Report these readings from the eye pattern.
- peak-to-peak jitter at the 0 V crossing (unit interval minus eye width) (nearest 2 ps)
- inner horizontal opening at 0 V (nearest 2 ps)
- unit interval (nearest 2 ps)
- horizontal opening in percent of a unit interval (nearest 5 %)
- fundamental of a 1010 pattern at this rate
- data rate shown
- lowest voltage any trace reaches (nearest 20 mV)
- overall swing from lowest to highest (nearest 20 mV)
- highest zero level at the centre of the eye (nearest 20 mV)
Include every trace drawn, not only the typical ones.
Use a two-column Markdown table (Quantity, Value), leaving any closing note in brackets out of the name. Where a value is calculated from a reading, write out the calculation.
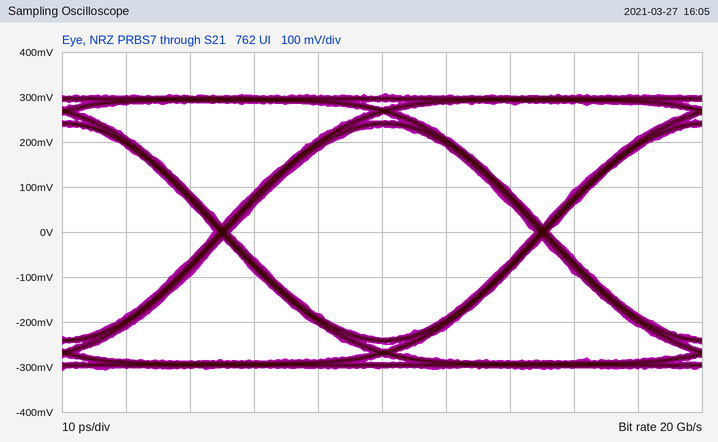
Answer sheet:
| Quantity | Value |
|---|---|
| peak-to-peak jitter at the 0 V crossing (unit interval minus eye width) | 2 ps |
| inner horizontal opening at 0 V | 48 ps |
| unit interval | 50 ps |
| horizontal opening in percent of a unit interval | 48 ps / 50 ps ≈ 96.0 %, so 95 % to the nearest 5 % |
| fundamental of a 1010 pattern at this rate | 10 GHz |
| data rate shown | 20 Gb/s |
| lowest voltage any trace reaches | -300 mV |
| overall swing from lowest to highest | 620 mV |
| highest zero level at the centre of the eye | -240 mV |
